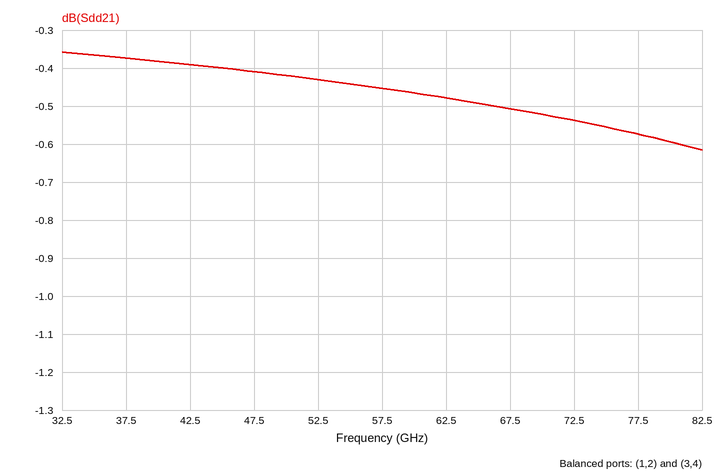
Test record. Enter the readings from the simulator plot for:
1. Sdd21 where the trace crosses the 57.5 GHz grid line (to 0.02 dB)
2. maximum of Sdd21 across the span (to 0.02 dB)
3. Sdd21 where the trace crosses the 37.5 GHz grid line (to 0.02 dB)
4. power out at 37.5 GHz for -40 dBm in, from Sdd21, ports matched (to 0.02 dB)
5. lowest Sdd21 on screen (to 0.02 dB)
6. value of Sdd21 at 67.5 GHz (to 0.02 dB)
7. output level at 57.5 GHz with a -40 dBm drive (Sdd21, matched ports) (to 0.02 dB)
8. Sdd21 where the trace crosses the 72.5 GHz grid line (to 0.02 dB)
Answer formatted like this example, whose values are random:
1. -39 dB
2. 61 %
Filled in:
1. -0.46 dB
2. -0.36 dB
3. -0.38 dB
4. -40.38 dBm
5. -0.62 dB
6. -0.50 dB
7. -40.46 dBm
8. -0.54 dB
